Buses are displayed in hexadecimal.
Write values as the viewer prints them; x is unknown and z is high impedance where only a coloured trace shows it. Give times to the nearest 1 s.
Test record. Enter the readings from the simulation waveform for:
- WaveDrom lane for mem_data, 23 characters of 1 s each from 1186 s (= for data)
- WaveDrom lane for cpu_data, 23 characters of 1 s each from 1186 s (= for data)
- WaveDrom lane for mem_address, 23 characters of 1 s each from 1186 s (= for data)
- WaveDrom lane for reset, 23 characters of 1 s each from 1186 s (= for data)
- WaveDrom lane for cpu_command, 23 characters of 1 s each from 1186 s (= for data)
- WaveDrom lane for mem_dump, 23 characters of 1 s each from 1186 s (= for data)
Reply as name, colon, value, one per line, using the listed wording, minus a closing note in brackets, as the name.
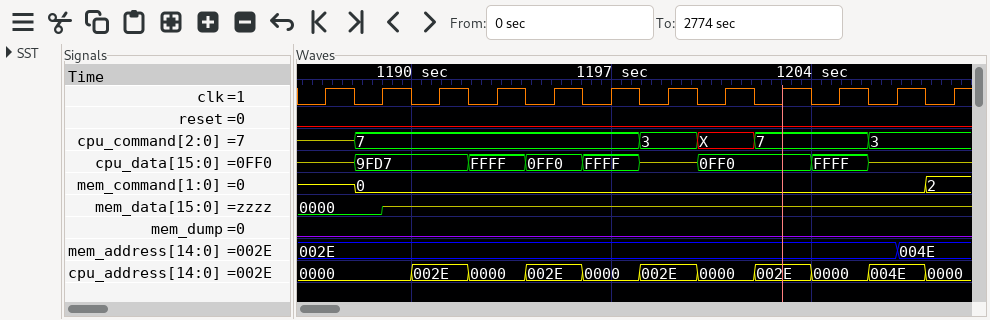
WaveDrom lane for mem_data, 23 characters of 1 s each from 1186 s: {name: 'mem_data', wave: '=..z...................', data: '0000'}
WaveDrom lane for cpu_data, 23 characters of 1 s each from 1186 s: {name: 'cpu_data', wave: 'z.=...=.=.=.z.=...=.z..', data: '9FD7 FFFF 0FF0 FFFF 0FF0 FFFF'}
WaveDrom lane for mem_address, 23 characters of 1 s each from 1186 s: {name: 'mem_address', wave: '=....................=.', data: '002E 004E'}
WaveDrom lane for reset, 23 characters of 1 s each from 1186 s: {name: 'reset', wave: '0......................'}
WaveDrom lane for cpu_command, 23 characters of 1 s each from 1186 s: {name: 'cpu_command', wave: 'z.=.........=.=.=...=..', data: '7 3 X 7 3'}
WaveDrom lane for mem_dump, 23 characters of 1 s each from 1186 s: {name: 'mem_dump', wave: '0......................'}
